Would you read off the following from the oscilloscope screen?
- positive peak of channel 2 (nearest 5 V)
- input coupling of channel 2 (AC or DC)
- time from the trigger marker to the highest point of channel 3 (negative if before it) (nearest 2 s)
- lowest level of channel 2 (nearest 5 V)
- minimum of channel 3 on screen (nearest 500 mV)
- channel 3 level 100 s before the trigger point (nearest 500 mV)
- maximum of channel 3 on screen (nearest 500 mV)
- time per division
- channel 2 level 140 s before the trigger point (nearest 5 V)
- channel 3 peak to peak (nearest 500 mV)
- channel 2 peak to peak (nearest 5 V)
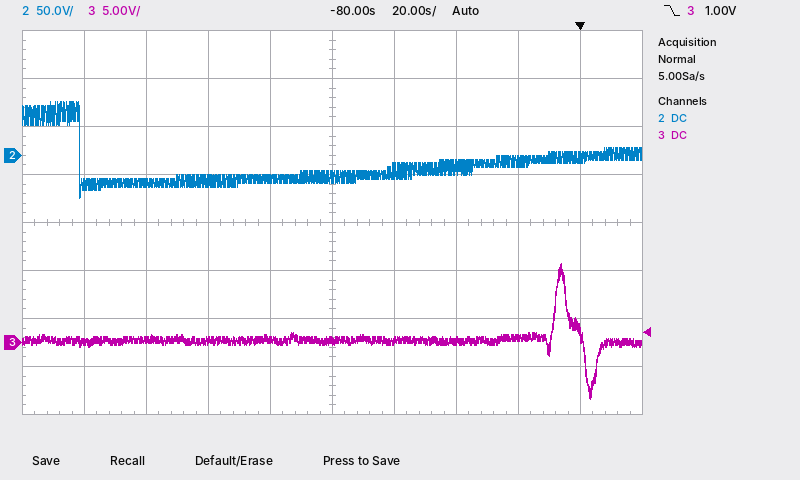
55 V
DC
-6 s
-45 V
-6.0 V
500 mV
8.0 V
20 s
-30 V
14.0 V
100 V
